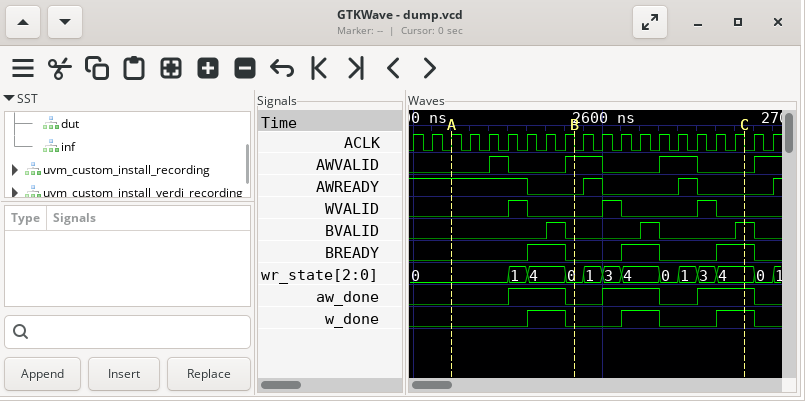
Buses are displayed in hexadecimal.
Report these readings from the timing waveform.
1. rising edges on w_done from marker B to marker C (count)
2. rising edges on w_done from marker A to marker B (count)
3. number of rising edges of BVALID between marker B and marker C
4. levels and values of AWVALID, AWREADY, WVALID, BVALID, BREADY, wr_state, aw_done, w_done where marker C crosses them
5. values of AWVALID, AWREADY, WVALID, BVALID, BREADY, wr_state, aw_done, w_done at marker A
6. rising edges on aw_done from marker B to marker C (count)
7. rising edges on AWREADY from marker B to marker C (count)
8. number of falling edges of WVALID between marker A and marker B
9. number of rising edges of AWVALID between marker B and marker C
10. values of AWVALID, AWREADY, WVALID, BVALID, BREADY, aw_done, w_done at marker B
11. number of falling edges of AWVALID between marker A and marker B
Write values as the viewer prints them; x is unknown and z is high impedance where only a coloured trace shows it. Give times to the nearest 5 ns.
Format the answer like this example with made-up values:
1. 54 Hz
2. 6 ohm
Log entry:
1. 2
2. 1
3. 2
4. AWVALID=0, AWREADY=0, WVALID=0, BVALID=1, BREADY=1, wr_state=4, aw_done=1, w_done=1
5. AWVALID=0, AWREADY=1, WVALID=0, BVALID=0, BREADY=0, wr_state=0, aw_done=0, w_done=0
6. 2
7. 2
8. 1
9. 1
10. AWVALID=1, AWREADY=0, WVALID=0, BVALID=0, BREADY=0, aw_done=0, w_done=0
11. 1
